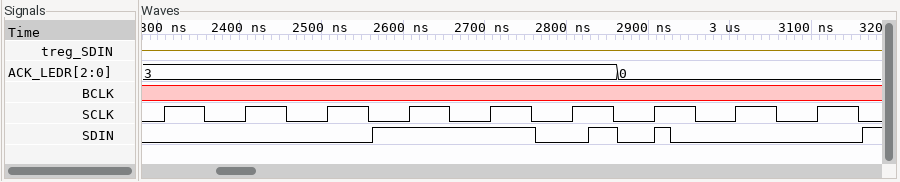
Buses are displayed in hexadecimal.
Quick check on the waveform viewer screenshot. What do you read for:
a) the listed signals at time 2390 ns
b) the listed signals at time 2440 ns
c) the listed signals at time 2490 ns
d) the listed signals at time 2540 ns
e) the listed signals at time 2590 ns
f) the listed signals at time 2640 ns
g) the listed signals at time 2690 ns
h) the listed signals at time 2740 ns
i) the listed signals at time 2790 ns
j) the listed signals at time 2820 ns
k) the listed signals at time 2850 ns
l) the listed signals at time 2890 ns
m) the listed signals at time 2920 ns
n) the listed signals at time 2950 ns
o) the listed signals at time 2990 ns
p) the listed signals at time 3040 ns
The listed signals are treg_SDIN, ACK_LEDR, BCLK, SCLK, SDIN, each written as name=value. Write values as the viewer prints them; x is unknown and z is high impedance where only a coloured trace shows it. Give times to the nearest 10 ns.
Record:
treg_SDIN=z, ACK_LEDR=3, BCLK=x, SCLK=0, SDIN=0
treg_SDIN=z, ACK_LEDR=3, BCLK=x, SCLK=1, SDIN=0
treg_SDIN=z, ACK_LEDR=3, BCLK=x, SCLK=0, SDIN=0
treg_SDIN=z, ACK_LEDR=3, BCLK=x, SCLK=1, SDIN=0
treg_SDIN=z, ACK_LEDR=3, BCLK=x, SCLK=0, SDIN=1
treg_SDIN=z, ACK_LEDR=3, BCLK=x, SCLK=1, SDIN=1
treg_SDIN=z, ACK_LEDR=3, BCLK=x, SCLK=0, SDIN=1
treg_SDIN=z, ACK_LEDR=3, BCLK=x, SCLK=1, SDIN=1
treg_SDIN=z, ACK_LEDR=3, BCLK=x, SCLK=0, SDIN=0
treg_SDIN=z, ACK_LEDR=3, BCLK=x, SCLK=1, SDIN=0
treg_SDIN=z, ACK_LEDR=3, BCLK=x, SCLK=1, SDIN=1
treg_SDIN=z, ACK_LEDR=0, BCLK=x, SCLK=0, SDIN=0
treg_SDIN=z, ACK_LEDR=0, BCLK=x, SCLK=1, SDIN=1
treg_SDIN=z, ACK_LEDR=0, BCLK=x, SCLK=1, SDIN=0
treg_SDIN=z, ACK_LEDR=0, BCLK=x, SCLK=0, SDIN=0
treg_SDIN=z, ACK_LEDR=0, BCLK=x, SCLK=1, SDIN=0
